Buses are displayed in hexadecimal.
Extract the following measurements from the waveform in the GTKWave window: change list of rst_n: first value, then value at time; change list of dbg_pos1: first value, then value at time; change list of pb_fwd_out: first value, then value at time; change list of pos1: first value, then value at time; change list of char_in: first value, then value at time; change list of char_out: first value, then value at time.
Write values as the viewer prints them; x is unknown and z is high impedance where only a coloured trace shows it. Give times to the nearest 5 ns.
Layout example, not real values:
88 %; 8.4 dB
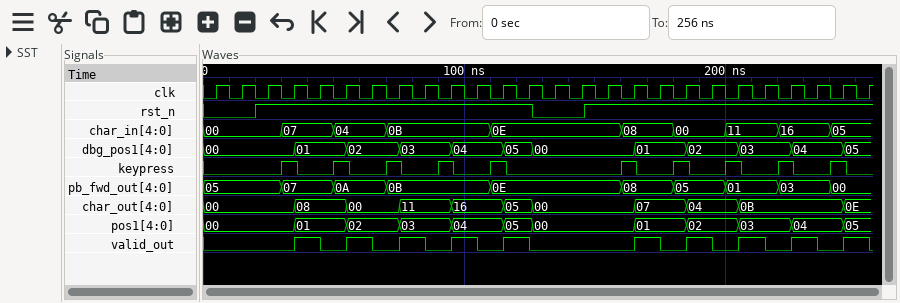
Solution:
0, 1 at 20 ns, 0 at 125 ns, 1 at 145 ns; 00, 01 at 35 ns, 02 at 55 ns, 03 at 75 ns, 04 at 95 ns, 05 at 115 ns, 00 at 125 ns, 01 at 165 ns, 02 at 185 ns, 03 at 205 ns, 04 at 225 ns, 05 at 245 ns; 05, 07 at 30 ns, 0A at 50 ns, 0B at 70 ns, 0E at 110 ns, 08 at 160 ns, 05 at 180 ns, 01 at 200 ns, 03 at 220 ns, 00 at 240 ns; 00, 01 at 35 ns, 02 at 55 ns, 03 at 75 ns, 04 at 95 ns, 05 at 115 ns, 00 at 125 ns, 01 at 165 ns, 02 at 185 ns, 03 at 205 ns, 04 at 225 ns, 05 at 245 ns; 00, 07 at 30 ns, 04 at 50 ns, 0B at 70 ns, 0E at 110 ns, 08 at 160 ns, 00 at 180 ns, 11 at 200 ns, 16 at 220 ns, 05 at 240 ns; 00, 08 at 35 ns, 00 at 55 ns, 11 at 75 ns, 16 at 95 ns, 05 at 115 ns, 00 at 125 ns, 07 at 165 ns, 04 at 185 ns, 0B at 205 ns, 0E at 245 ns
